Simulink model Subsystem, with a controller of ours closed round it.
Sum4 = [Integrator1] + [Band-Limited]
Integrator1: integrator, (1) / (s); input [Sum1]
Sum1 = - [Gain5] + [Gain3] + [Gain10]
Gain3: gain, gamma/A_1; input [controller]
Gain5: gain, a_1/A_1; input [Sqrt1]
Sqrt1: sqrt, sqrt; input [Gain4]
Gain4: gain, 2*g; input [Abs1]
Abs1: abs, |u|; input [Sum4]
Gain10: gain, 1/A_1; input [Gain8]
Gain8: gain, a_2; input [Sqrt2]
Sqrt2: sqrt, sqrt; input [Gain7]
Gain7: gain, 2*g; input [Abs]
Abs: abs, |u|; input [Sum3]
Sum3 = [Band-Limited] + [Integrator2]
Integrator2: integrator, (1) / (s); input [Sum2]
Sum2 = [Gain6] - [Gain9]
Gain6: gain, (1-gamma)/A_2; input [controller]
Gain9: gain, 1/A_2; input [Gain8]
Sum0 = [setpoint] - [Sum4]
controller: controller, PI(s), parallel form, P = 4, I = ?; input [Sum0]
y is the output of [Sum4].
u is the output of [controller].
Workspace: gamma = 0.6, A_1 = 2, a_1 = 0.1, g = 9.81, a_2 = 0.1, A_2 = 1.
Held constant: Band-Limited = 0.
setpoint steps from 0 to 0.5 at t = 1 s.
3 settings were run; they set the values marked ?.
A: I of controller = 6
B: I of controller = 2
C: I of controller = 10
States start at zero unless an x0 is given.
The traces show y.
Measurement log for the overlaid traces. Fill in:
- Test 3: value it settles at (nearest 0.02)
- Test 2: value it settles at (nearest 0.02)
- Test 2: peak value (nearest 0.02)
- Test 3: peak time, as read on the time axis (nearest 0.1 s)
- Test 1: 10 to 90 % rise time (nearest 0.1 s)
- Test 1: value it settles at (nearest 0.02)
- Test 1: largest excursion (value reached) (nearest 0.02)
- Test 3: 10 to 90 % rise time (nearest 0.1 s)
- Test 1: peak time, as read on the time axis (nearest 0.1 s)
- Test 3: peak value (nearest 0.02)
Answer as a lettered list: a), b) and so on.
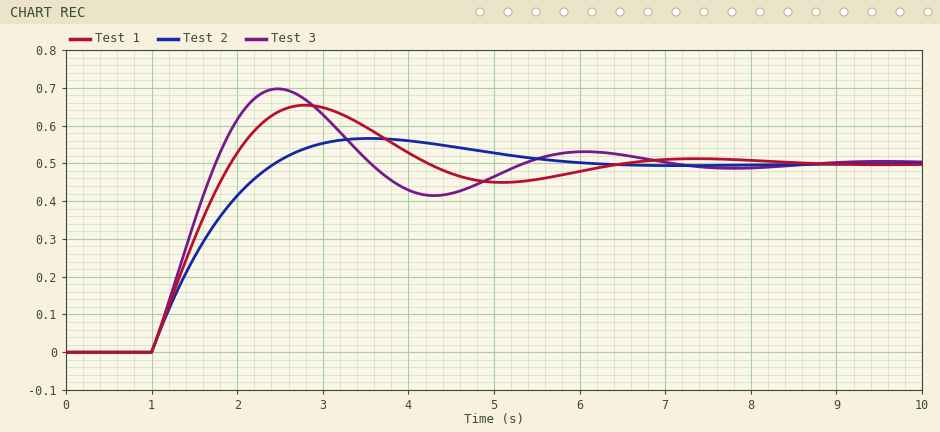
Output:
a) 0.50
b) 0.50
c) 0.56
d) 2.5 s
e) 0.7 s
f) 0.50
g) 0.66
h) 0.6 s
i) 2.8 s
j) 0.70
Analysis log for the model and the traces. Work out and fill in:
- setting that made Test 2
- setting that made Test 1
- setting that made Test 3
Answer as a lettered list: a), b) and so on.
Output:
a) B
b) A
c) C
